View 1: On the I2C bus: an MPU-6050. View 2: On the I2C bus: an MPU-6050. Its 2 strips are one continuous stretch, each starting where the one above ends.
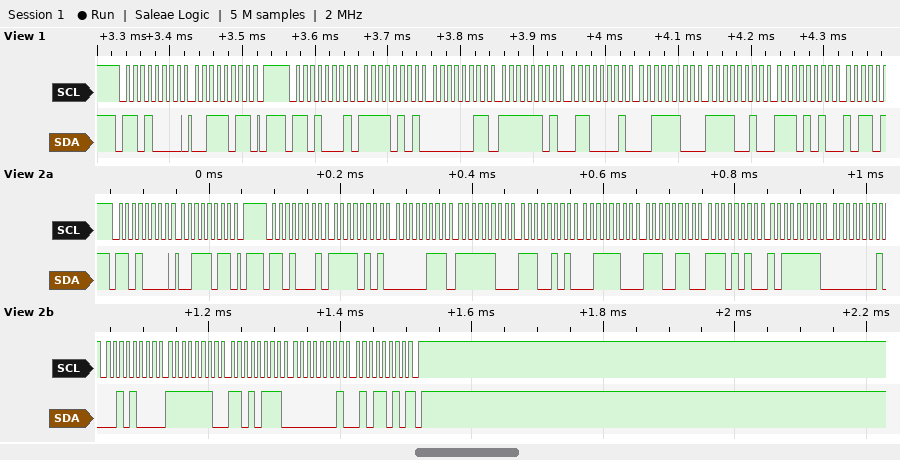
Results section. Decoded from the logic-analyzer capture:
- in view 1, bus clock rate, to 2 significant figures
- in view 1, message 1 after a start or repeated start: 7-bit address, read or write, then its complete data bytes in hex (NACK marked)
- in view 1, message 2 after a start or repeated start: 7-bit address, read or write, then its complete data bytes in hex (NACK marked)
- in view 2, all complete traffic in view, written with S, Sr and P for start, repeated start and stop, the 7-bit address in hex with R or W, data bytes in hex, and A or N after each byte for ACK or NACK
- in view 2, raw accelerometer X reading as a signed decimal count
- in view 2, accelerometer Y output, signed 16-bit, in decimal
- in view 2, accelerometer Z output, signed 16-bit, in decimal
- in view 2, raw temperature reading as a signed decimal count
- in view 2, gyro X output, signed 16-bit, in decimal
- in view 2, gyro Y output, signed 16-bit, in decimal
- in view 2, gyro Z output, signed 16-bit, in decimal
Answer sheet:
100 kHz
0x68 write: 3B
0x68 read: F5 03 FD 61 3C F2 EA
S 68W A 3B A P S 68R A F5 A 07 A FC A E5 A 3C A E6 A EA A BF A 01 A 28 A FE A D7 A 01 A 5A N P
-2809
-795
15590
-5441
296
-297
346
